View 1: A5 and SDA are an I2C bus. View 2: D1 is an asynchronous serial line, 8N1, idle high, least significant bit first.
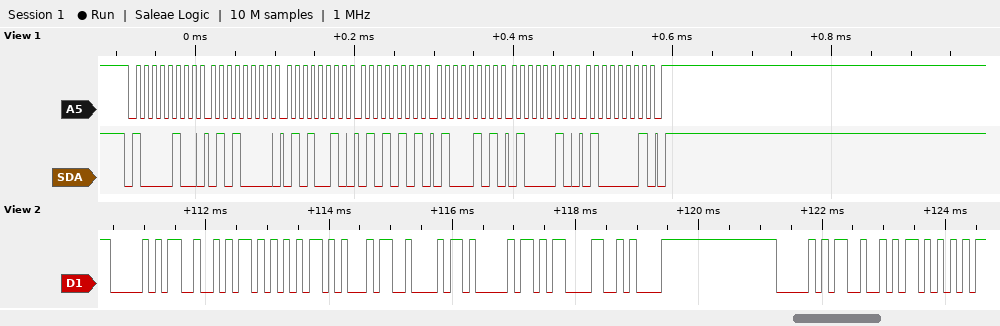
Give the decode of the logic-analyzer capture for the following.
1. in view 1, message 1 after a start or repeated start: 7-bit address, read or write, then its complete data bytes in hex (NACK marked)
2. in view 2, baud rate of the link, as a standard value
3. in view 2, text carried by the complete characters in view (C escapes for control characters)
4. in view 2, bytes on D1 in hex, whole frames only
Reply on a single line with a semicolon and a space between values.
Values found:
0x42 write: 50 52 55 45 42 41; 9600 baud; "PRUEBA\r\nPRU"; 0x50 0x52 0x55 0x45 0x42 0x41 0x0D 0x0A 0x50 0x52 0x55
